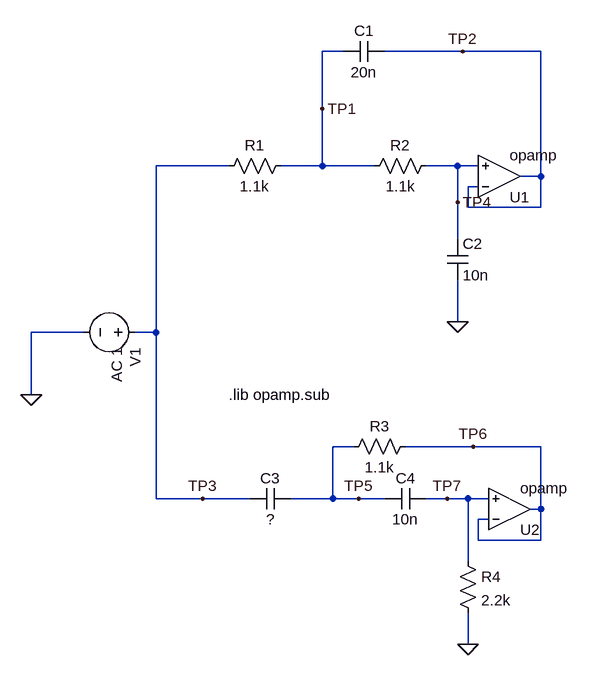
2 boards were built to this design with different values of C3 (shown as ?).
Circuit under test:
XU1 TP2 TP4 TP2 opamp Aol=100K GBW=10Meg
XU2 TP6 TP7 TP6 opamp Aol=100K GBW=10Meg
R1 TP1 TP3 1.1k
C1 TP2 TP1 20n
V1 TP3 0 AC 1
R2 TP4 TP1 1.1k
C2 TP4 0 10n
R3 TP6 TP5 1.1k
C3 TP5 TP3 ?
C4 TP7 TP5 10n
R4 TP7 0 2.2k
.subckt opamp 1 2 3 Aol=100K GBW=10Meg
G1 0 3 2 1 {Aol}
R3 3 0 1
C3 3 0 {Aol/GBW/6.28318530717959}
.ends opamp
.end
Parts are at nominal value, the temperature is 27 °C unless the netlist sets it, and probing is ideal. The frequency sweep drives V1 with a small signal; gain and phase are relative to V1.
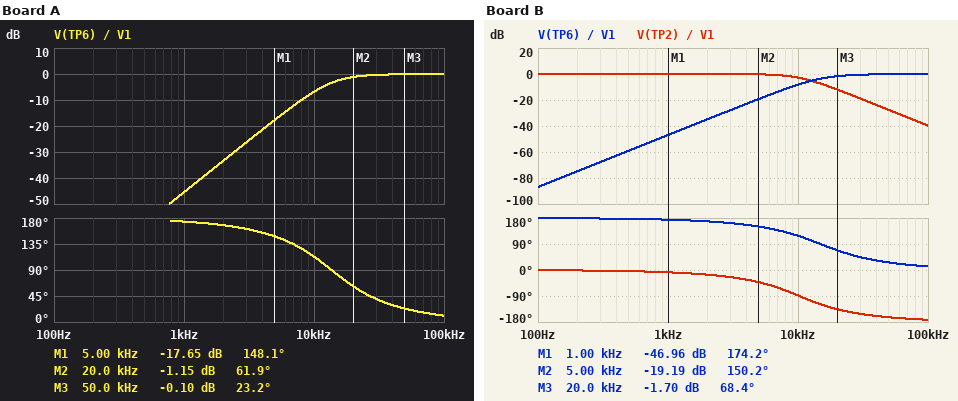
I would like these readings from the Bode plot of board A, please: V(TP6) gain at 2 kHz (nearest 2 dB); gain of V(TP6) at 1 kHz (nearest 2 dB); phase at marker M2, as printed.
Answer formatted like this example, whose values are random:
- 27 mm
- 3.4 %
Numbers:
- -34 dB
- -46 dB
- 61.9 deg
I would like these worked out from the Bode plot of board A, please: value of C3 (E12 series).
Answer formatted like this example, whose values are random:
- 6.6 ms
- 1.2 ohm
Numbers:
- 5.6 nF
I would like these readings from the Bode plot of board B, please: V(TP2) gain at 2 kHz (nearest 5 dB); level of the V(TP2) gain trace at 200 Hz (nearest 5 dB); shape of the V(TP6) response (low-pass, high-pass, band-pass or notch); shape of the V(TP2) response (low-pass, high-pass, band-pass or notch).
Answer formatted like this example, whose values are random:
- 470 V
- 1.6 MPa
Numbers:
- 0 dB
- 0 dB
- high-pass
- low-pass
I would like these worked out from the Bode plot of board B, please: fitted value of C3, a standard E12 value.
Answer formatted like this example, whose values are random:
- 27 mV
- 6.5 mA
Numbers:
- 4.7 nF
